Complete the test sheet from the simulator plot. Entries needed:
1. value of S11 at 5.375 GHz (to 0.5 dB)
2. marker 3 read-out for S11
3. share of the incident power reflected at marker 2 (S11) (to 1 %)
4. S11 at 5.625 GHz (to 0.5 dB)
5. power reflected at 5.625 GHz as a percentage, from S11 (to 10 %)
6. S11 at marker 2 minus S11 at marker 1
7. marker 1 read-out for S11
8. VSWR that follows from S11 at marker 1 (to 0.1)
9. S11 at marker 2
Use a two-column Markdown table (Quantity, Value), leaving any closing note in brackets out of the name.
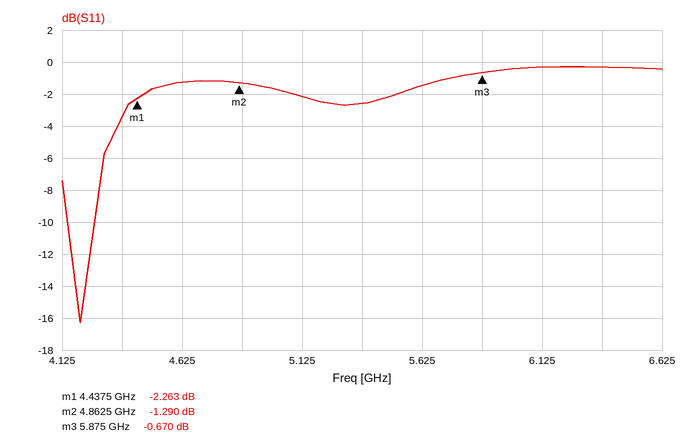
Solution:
| Quantity | Value |
|---|---|
| value of S11 at 5.375 GHz | -2.5 dB |
| marker 3 read-out for S11 | -0.670 dB |
| share of the incident power reflected at marker 2 (S11) | 74 % |
| S11 at 5.625 GHz | -1.5 dB |
| power reflected at 5.625 GHz as a percentage, from S11 | 70 % |
| S11 at marker 2 minus S11 at marker 1 | 0.973 dB |
| marker 1 read-out for S11 | -2.263 dB |
| VSWR that follows from S11 at marker 1 | 7.7 |
| S11 at marker 2 | -1.290 dB |
